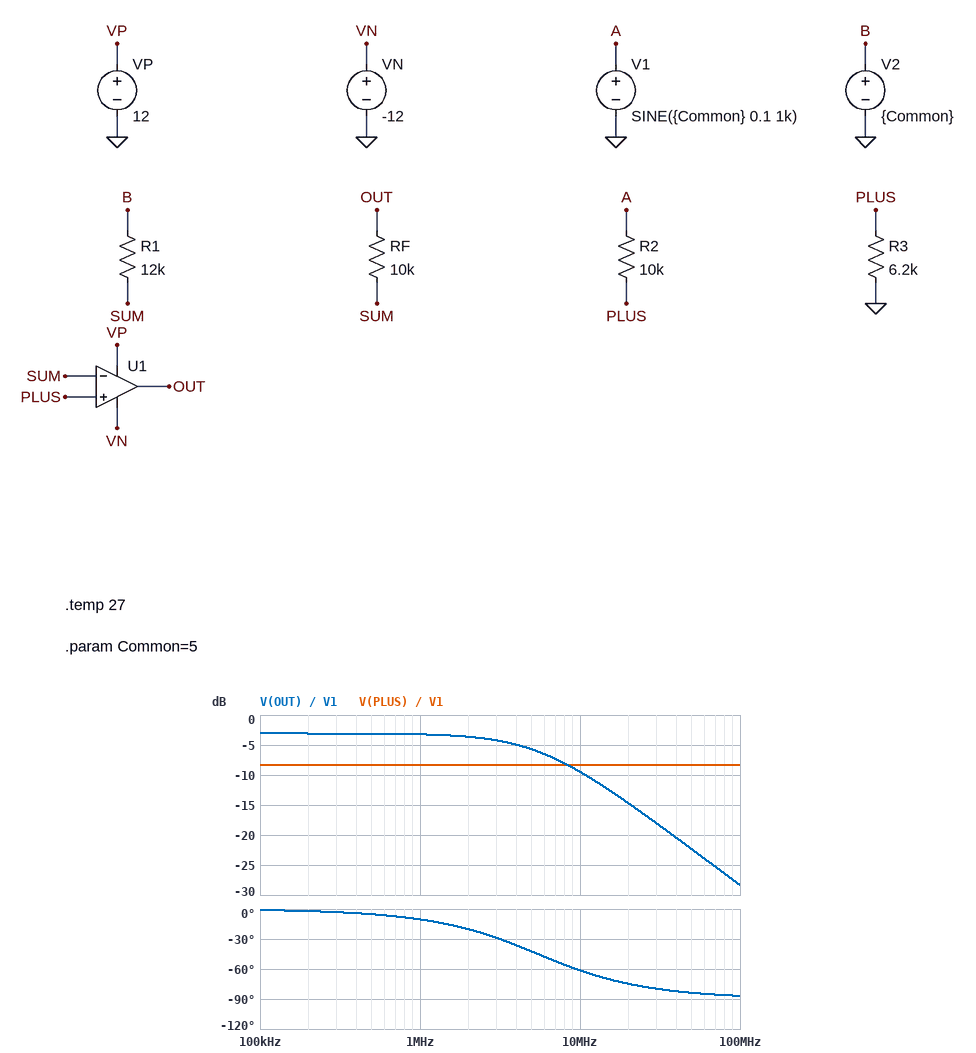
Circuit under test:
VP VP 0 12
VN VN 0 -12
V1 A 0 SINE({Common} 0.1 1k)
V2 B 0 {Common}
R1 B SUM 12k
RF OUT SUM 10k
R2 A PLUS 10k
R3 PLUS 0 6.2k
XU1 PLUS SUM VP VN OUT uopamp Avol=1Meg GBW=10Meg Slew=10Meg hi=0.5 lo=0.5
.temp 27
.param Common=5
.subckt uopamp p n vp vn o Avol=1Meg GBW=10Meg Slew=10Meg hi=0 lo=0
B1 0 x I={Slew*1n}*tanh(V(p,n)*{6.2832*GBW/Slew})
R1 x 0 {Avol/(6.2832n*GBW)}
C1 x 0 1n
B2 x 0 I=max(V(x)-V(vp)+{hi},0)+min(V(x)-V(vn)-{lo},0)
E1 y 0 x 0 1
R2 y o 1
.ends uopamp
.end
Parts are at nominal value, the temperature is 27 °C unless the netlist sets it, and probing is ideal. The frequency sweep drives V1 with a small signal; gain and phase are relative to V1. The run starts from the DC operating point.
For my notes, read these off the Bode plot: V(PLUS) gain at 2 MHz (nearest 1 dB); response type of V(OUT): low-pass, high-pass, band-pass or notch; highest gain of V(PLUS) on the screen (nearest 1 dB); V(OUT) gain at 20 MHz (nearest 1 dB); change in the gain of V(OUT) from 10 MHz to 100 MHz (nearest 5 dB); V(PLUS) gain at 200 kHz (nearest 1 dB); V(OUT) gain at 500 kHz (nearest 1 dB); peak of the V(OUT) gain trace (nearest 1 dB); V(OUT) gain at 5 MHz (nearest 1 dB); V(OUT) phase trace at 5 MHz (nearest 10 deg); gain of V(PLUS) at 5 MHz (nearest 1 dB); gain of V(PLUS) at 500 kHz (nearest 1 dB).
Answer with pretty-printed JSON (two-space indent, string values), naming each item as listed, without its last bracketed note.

{
  "V(PLUS) gain at 2 MHz": "-8 dB",
  "response type of V(OUT): low-pass, high-pass, band-pass or notch": "low-pass",
  "highest gain of V(PLUS) on the screen": "-8 dB",
  "V(OUT) gain at 20 MHz": "-15 dB",
  "change in the gain of V(OUT) from 10 MHz to 100 MHz": "-20 dB",
  "V(PLUS) gain at 200 kHz": "-8 dB",
  "V(OUT) gain at 500 kHz": "-3 dB",
  "peak of the V(OUT) gain trace": "-3 dB",
  "V(OUT) gain at 5 MHz": "-6 dB",
  "V(OUT) phase trace at 5 MHz": "-40 deg",
  "gain of V(PLUS) at 5 MHz": "-8 dB",
  "gain of V(PLUS) at 500 kHz": "-8 dB"
}
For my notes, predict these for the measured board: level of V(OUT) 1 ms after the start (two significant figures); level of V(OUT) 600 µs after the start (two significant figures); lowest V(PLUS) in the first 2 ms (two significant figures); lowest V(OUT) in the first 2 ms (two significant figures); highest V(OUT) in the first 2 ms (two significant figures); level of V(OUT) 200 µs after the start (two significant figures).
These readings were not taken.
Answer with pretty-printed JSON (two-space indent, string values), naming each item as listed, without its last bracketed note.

{
  "level of V(OUT) 1 ms after the start": "-660 mV",
  "level of V(OUT) 600 µs after the start": "-700 mV",
  "lowest V(PLUS) in the first 2 ms": "1.9 V",
  "lowest V(OUT) in the first 2 ms": "-730 mV",
  "highest V(OUT) in the first 2 ms": "-590 mV",
  "level of V(OUT) 200 µs after the start": "-590 mV"
}
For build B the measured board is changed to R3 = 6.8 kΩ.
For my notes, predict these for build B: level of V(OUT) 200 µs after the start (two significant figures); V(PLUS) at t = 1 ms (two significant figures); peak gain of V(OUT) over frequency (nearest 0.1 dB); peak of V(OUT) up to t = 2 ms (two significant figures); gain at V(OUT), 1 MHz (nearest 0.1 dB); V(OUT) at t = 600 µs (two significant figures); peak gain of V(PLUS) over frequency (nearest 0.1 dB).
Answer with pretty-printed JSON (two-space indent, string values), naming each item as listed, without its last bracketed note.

{
  "level of V(OUT) 200 µs after the start": "-390 mV",
  "V(PLUS) at t = 1 ms": "2.0 V",
  "peak gain of V(OUT) over frequency": "-2.6 dB",
  "peak of V(OUT) up to t = 2 ms": "-380 mV",
  "gain at V(OUT), 1 MHz": "-2.7 dB",
  "V(OUT) at t = 600 µs": "-500 mV",
  "peak gain of V(PLUS) over frequency": "-7.9 dB"
}
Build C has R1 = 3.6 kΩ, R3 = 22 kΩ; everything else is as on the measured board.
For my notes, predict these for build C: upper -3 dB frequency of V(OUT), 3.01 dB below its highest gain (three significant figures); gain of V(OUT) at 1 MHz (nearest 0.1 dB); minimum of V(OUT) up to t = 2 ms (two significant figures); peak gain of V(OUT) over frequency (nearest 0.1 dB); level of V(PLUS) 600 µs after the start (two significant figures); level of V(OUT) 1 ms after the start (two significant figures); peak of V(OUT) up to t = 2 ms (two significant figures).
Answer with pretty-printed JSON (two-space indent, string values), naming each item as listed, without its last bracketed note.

{
  "upper -3 dB frequency of V(OUT), 3.01 dB below its highest gain": "2.65 MHz",
  "gain of V(OUT) at 1 MHz": "7.7 dB",
  "minimum of V(OUT) up to t = 2 ms": "-1.2 V",
  "peak gain of V(OUT) over frequency": "8.3 dB",
  "level of V(PLUS) 600 µs after the start": "3.4 V",
  "level of V(OUT) 1 ms after the start": "-900 mV",
  "peak of V(OUT) up to t = 2 ms": "-640 mV"
}
